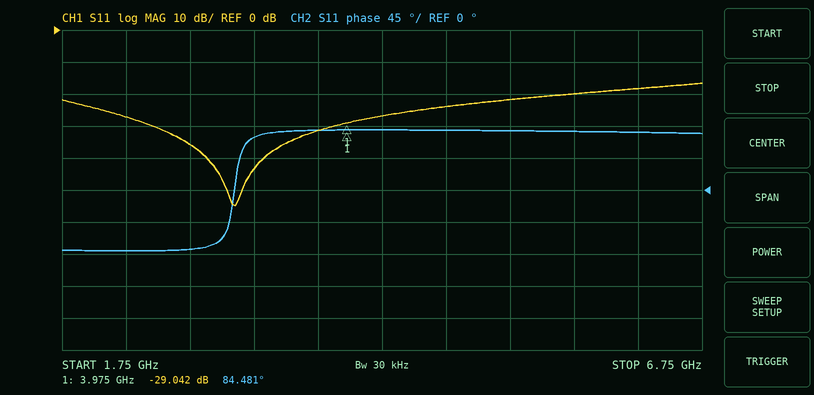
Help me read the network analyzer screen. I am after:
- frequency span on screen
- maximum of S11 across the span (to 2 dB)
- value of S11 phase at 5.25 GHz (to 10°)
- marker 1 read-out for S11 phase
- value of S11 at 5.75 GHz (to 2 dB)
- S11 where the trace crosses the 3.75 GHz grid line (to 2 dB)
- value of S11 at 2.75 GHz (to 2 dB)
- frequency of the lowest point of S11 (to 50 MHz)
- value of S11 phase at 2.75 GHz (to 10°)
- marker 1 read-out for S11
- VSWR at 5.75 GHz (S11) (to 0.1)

5 GHz
-16 dB
80°
84.481°
-20 dB
-32 dB
-36 dB
3.10 GHz
-80°
-29.042 dB
1.2
